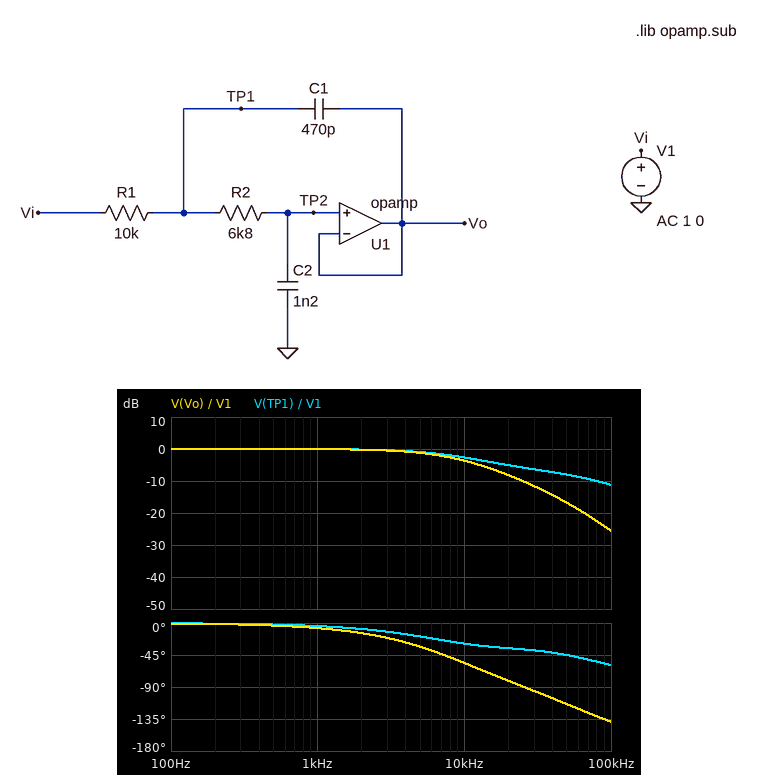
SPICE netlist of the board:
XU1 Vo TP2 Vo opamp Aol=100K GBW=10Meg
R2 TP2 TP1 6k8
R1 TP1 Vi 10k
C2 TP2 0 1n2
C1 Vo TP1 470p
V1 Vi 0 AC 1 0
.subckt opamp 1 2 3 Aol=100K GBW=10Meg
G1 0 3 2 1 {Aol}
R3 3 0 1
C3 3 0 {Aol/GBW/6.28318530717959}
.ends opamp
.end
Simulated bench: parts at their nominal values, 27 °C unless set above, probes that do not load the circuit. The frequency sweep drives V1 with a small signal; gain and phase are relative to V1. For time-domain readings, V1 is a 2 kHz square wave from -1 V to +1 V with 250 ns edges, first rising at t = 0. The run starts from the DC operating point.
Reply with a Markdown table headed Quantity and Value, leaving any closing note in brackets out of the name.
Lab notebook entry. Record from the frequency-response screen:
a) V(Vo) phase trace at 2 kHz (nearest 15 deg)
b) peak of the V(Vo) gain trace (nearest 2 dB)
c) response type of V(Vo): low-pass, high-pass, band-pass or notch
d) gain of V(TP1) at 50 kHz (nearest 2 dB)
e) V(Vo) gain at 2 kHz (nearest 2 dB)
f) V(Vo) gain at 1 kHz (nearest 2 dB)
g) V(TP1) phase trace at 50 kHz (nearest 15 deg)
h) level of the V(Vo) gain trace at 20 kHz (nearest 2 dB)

| Quantity | Value |
|---|---|
| V(Vo) phase trace at 2 kHz | -15 deg |
| peak of the V(Vo) gain trace | 0 dB |
| response type of V(Vo): low-pass, high-pass, band-pass or notch | low-pass |
| gain of V(TP1) at 50 kHz | -8 dB |
| V(Vo) gain at 2 kHz | 0 dB |
| V(Vo) gain at 1 kHz | 0 dB |
| V(TP1) phase trace at 50 kHz | -45 deg |
| level of the V(Vo) gain trace at 20 kHz | -8 dB |
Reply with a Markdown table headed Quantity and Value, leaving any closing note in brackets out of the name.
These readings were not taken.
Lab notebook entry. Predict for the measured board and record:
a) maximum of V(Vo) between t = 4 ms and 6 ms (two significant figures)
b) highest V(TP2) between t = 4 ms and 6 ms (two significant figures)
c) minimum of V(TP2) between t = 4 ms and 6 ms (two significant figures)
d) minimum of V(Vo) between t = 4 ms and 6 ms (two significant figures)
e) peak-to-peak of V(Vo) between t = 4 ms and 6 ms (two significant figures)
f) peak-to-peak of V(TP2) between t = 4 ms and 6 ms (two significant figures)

| Quantity | Value |
|---|---|
| maximum of V(Vo) between t = 4 ms and 6 ms | 1.0 V |
| highest V(TP2) between t = 4 ms and 6 ms | 1.0 V |
| minimum of V(TP2) between t = 4 ms and 6 ms | -1.0 V |
| minimum of V(Vo) between t = 4 ms and 6 ms | -1.0 V |
| peak-to-peak of V(Vo) between t = 4 ms and 6 ms | 2.0 V |
| peak-to-peak of V(TP2) between t = 4 ms and 6 ms | 2.0 V |
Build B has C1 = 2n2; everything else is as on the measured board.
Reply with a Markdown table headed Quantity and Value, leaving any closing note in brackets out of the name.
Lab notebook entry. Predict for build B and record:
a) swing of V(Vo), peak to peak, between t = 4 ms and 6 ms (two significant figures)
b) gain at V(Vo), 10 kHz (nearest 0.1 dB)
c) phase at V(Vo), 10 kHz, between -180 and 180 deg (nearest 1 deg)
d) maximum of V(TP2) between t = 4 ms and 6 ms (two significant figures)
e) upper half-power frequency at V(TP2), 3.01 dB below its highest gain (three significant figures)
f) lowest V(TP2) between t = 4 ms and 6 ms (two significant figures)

| Quantity | Value |
|---|---|
| swing of V(Vo), peak to peak, between t = 4 ms and 6 ms | 2.1 V |
| gain at V(Vo), 10 kHz | -2.3 dB |
| phase at V(Vo), 10 kHz, between -180 and 180 deg | -77 deg |
| maximum of V(TP2) between t = 4 ms and 6 ms | 1.1 V |
| upper half-power frequency at V(TP2), 3.01 dB below its highest gain | 11.1 kHz |
| lowest V(TP2) between t = 4 ms and 6 ms | -1.1 V |
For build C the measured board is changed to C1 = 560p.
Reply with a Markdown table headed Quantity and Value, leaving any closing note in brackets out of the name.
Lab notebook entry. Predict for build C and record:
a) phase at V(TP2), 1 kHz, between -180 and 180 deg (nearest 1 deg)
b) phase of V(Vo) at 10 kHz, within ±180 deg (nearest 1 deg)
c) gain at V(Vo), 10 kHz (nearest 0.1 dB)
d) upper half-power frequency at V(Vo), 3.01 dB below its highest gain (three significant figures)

| Quantity | Value |
|---|---|
| phase at V(TP2), 1 kHz, between -180 and 180 deg | -7 deg |
| phase of V(Vo) at 10 kHz, within ±180 deg | -57 deg |
| gain at V(Vo), 10 kHz | -3.6 dB |
| upper half-power frequency at V(Vo), 3.01 dB below its highest gain | 8.88 kHz |
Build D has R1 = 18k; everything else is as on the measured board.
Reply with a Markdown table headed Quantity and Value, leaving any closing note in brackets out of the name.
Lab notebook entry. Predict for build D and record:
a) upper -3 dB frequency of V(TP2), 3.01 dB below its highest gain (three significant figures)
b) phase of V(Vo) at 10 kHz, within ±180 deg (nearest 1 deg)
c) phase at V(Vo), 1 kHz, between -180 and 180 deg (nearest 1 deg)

| Quantity | Value |
|---|---|
| upper -3 dB frequency of V(TP2), 3.01 dB below its highest gain | 5.80 kHz |
| phase of V(Vo) at 10 kHz, within ±180 deg | -69 deg |
| phase at V(Vo), 1 kHz, between -180 and 180 deg | -11 deg |
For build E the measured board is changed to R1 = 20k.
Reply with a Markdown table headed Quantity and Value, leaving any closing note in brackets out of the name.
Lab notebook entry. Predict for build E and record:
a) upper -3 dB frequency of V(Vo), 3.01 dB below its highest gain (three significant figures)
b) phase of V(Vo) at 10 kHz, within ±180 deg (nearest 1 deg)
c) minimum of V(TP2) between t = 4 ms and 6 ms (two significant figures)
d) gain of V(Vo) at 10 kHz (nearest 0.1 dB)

| Quantity | Value |
|---|---|
| upper -3 dB frequency of V(Vo), 3.01 dB below its highest gain | 5.34 kHz |
| phase of V(Vo) at 10 kHz, within ±180 deg | -71 deg |
| minimum of V(TP2) between t = 4 ms and 6 ms | -1.0 V |
| gain of V(Vo) at 10 kHz | -6.6 dB |
